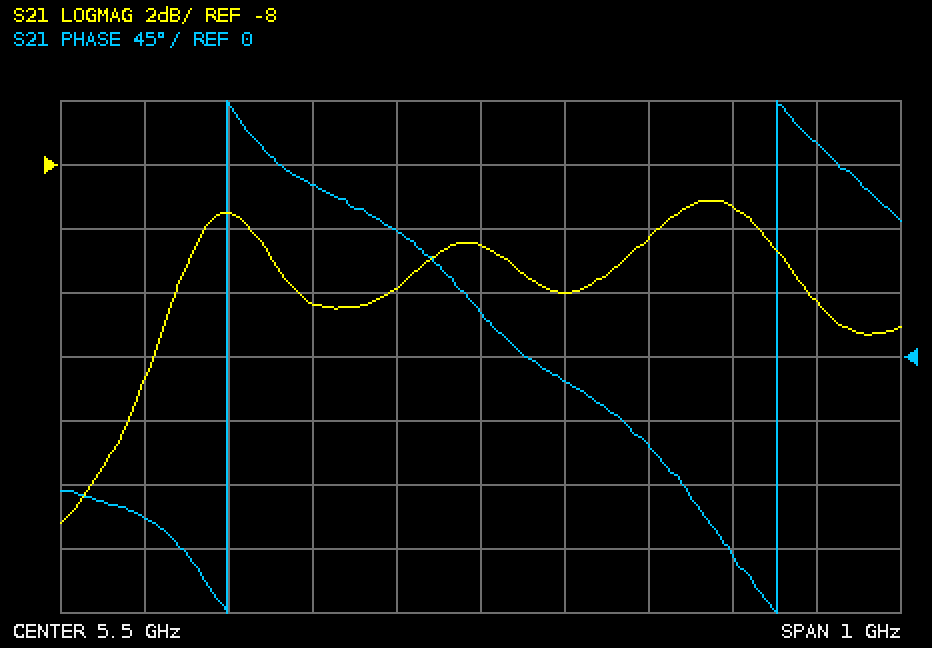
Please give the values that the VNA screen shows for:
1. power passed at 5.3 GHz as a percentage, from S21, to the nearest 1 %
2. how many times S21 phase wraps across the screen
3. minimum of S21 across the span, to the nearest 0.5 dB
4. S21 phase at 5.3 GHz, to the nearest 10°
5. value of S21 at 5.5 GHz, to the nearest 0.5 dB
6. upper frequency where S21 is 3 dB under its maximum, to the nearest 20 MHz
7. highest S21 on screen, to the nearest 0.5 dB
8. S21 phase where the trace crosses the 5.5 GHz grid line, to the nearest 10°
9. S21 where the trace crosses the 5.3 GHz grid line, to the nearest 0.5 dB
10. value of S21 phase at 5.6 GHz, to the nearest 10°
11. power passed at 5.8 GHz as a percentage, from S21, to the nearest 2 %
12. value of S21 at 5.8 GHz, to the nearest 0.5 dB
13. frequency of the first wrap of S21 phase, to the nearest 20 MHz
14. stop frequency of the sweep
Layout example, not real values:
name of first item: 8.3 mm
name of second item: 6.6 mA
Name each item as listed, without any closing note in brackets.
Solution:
power passed at 5.3 GHz as a percentage, from S21, to the nearest 1 %: 6 %
how many times S21 phase wraps across the screen: 2
minimum of S21 across the span, to the nearest 0.5 dB: -19.0 dB
S21 phase at 5.3 GHz, to the nearest 10°: 120°
value of S21 at 5.5 GHz, to the nearest 0.5 dB: -10.5 dB
upper frequency where S21 is 3 dB under its maximum, to the nearest 20 MHz: 5.90 GHz
highest S21 on screen, to the nearest 0.5 dB: -9.0 dB
S21 phase where the trace crosses the 5.5 GHz grid line, to the nearest 10°: 30°
S21 where the trace crosses the 5.3 GHz grid line, to the nearest 0.5 dB: -12.5 dB
value of S21 phase at 5.6 GHz, to the nearest 10°: -20°
power passed at 5.8 GHz as a percentage, from S21, to the nearest 2 %: 12 %
value of S21 at 5.8 GHz, to the nearest 0.5 dB: -9.5 dB
frequency of the first wrap of S21 phase, to the nearest 20 MHz: 5.20 GHz
stop frequency of the sweep: 6 GHz
